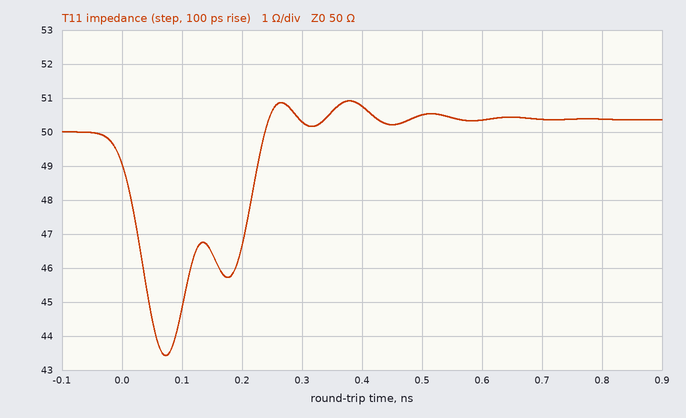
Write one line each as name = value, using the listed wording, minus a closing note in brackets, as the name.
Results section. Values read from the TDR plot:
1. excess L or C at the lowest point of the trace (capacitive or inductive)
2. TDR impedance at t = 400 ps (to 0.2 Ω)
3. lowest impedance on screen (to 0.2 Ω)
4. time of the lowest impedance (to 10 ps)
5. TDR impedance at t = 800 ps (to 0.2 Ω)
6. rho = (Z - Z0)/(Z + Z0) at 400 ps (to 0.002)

excess L or C at the lowest point of the trace = capacitive
TDR impedance at t = 400 ps = 50.8 Ω
lowest impedance on screen = 43.4 Ω
time of the lowest impedance = 70 ps
TDR impedance at t = 800 ps = 50.4 Ω
rho = (Z - Z0)/(Z + Z0) at 400 ps = +0.008
